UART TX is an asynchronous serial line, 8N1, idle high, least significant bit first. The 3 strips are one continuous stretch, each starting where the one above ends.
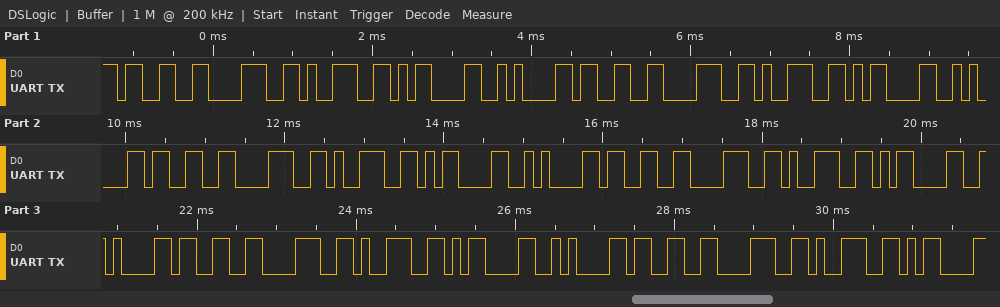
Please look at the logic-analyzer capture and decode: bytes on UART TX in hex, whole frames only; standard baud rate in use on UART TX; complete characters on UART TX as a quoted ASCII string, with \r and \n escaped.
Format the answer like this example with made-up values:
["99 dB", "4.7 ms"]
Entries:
["33 38 39 0D 0A 33 38 39 0D 0A 33 38 39 0D 0A 33 38 39 0D 0A 33 38 39 0D 0A 33 38 39 0D", "9600 baud", "\"389\\r\\n389\\r\\n389\\r\\n389\\r\\n389\\r\\n389\\r\""]
